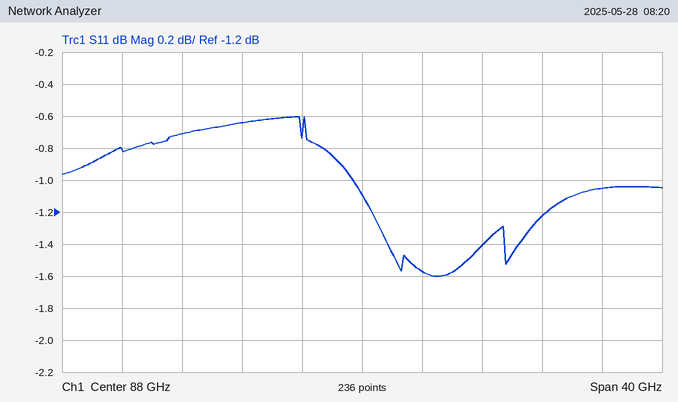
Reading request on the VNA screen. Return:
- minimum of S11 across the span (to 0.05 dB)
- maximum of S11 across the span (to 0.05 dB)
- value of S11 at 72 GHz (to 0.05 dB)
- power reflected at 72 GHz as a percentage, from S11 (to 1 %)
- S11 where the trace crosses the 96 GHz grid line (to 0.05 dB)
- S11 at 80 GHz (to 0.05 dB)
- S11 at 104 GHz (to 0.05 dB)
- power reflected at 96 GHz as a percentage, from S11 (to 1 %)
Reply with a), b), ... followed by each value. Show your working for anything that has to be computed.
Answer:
a) -1.60 dB
b) -0.60 dB
c) -0.80 dB
d) 10^(-0.8/10) ≈ 83 %
e) -1.40 dB
f) -0.65 dB
g) -1.05 dB
h) 10^(-1.4/10) ≈ 72 %
